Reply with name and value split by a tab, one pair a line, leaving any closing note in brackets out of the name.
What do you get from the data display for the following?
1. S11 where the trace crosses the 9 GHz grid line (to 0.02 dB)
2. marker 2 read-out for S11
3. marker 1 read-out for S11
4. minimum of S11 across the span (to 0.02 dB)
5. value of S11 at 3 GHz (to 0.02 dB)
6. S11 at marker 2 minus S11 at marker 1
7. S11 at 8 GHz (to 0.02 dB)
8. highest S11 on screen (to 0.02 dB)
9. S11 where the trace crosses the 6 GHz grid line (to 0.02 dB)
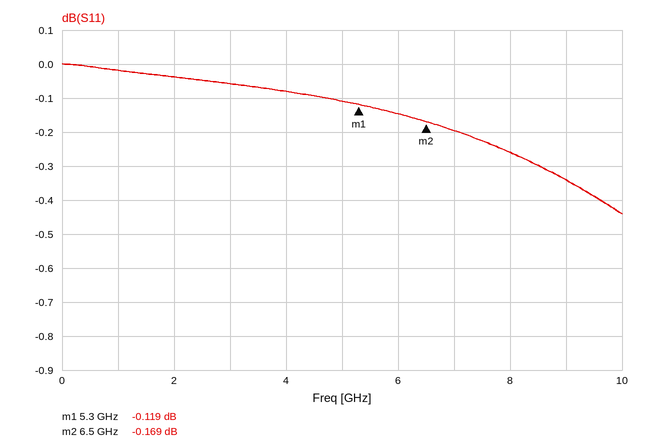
S11 where the trace crosses the 9 GHz grid line	-0.34 dB
marker 2 read-out for S11	-0.169 dB
marker 1 read-out for S11	-0.119 dB
minimum of S11 across the span	-0.44 dB
value of S11 at 3 GHz	-0.06 dB
S11 at marker 2 minus S11 at marker 1	-0.050 dB
S11 at 8 GHz	-0.26 dB
highest S11 on screen	0.00 dB
S11 where the trace crosses the 6 GHz grid line	-0.14 dB
